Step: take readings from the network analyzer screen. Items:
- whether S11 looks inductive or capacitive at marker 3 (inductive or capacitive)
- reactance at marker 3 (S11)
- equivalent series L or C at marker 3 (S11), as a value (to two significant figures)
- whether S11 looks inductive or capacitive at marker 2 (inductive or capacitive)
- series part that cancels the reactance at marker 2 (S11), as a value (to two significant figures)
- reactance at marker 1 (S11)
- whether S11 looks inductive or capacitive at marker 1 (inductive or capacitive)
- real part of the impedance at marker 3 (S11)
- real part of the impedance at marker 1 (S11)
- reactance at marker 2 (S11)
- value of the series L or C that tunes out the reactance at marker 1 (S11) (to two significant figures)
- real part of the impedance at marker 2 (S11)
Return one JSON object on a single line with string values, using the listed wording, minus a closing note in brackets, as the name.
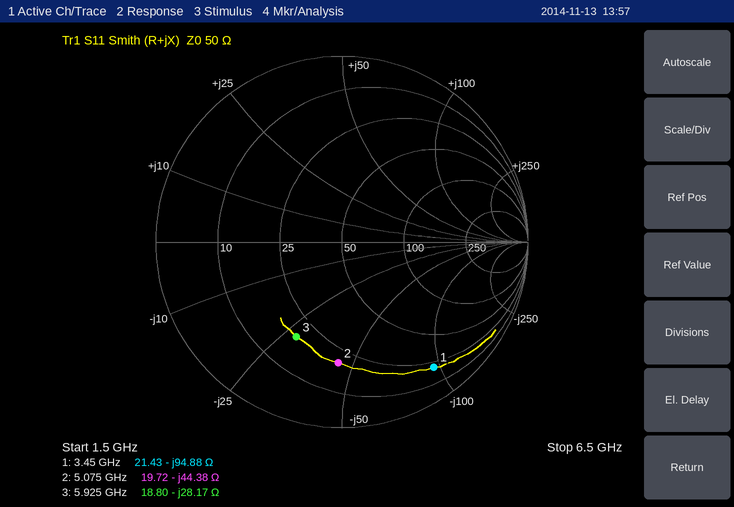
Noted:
{"whether S11 looks inductive or capacitive at marker 3": "capacitive", "reactance at marker 3": "-28.17 Ω", "equivalent series L or C at marker 3 (S11), as a value": "950 fF", "whether S11 looks inductive or capacitive at marker 2": "capacitive", "series part that cancels the reactance at marker 2 (S11), as a value": "1.4 nH", "reactance at marker 1": "-94.88 Ω", "whether S11 looks inductive or capacitive at marker 1": "capacitive", "real part of the impedance at marker 3": "18.80 Ω", "real part of the impedance at marker 1": "21.43 Ω", "reactance at marker 2": "-44.38 Ω", "value of the series L or C that tunes out the reactance at marker 1 (S11)": "4.4 nH", "real part of the impedance at marker 2": "19.72 Ω"}
